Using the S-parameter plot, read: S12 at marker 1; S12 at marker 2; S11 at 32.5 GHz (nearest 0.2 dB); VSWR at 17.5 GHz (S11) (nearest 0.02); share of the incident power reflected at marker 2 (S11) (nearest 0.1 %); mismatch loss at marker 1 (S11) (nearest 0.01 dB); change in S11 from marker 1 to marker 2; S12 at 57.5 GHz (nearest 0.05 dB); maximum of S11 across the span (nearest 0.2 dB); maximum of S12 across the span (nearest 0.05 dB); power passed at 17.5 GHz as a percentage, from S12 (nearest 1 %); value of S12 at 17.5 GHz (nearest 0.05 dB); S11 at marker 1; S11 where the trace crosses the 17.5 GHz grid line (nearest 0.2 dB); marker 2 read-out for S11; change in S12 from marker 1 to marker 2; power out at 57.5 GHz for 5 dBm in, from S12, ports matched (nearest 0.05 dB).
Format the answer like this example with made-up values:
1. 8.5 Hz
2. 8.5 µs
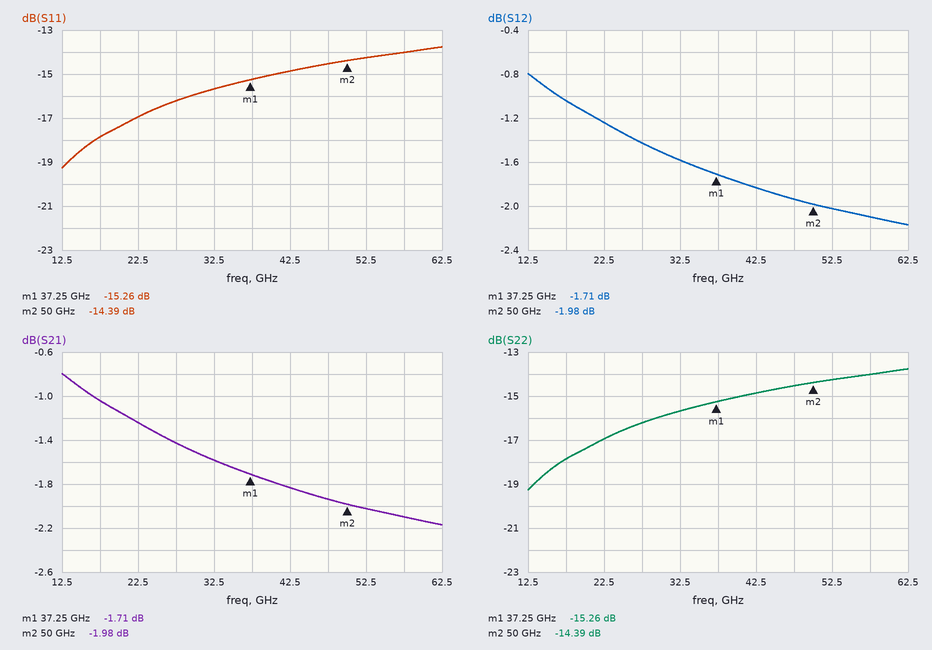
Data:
1. -1.71 dB
2. -1.98 dB
3. -15.6 dB
4. 1.30
5. 3.6 %
6. 0.13 dB
7. 0.87 dB
8. -2.10 dB
9. -13.8 dB
10. -0.80 dB
11. 79 %
12. -1.05 dB
13. -15.26 dB
14. -17.8 dB
15. -14.39 dB
16. -0.27 dB
17. 2.90 dBm
